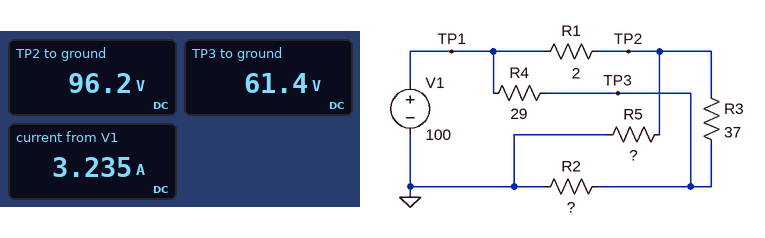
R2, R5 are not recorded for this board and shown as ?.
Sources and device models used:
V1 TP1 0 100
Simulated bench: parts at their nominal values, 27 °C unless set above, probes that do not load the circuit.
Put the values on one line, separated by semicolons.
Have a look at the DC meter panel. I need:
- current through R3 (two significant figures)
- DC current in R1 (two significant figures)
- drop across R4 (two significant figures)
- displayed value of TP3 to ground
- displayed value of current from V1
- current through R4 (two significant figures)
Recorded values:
940 mA; 1.9 A; 39 V; 61.4 V; 3.235 A; 1.3 A
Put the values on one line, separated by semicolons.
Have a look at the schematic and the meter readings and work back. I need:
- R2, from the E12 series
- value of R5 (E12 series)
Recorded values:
27 Ω; 100 Ω
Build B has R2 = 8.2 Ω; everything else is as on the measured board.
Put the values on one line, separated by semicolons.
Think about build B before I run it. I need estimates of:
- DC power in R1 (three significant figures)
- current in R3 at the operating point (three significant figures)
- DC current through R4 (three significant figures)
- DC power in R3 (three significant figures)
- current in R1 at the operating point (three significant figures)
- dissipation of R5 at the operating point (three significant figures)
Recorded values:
13.8 W; 1.68 A; 2.32 A; 104 W; 2.62 A; 89.8 W
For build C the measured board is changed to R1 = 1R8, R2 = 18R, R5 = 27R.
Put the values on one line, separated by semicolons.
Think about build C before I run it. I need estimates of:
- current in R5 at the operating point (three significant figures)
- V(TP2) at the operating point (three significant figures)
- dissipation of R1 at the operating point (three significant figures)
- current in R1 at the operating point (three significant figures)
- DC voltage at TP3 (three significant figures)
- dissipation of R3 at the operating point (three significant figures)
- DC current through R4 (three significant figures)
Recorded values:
3.40 A; 91.9 V; 36.7 W; 4.52 A; 50.7 V; 45.9 W; 1.70 A
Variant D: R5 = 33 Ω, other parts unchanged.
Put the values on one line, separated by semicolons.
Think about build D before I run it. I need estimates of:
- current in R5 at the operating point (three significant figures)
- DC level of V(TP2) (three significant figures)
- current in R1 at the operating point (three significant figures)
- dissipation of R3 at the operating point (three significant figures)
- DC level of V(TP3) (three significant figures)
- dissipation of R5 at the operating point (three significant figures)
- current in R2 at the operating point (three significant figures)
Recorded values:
2.81 A; 92.6 V; 3.68 A; 28.1 W; 60.4 V; 260 W; 2.24 A
